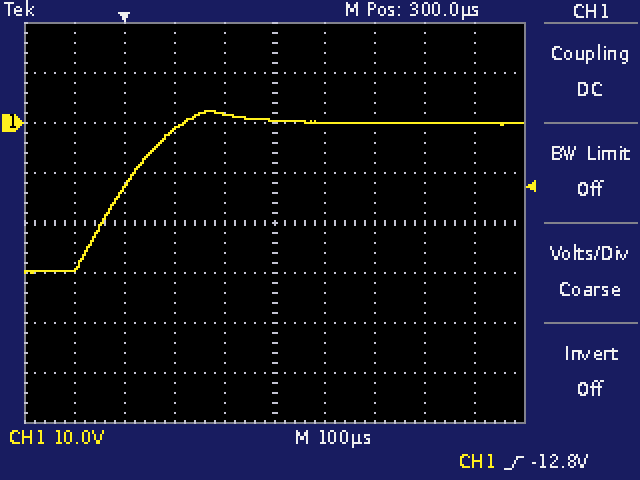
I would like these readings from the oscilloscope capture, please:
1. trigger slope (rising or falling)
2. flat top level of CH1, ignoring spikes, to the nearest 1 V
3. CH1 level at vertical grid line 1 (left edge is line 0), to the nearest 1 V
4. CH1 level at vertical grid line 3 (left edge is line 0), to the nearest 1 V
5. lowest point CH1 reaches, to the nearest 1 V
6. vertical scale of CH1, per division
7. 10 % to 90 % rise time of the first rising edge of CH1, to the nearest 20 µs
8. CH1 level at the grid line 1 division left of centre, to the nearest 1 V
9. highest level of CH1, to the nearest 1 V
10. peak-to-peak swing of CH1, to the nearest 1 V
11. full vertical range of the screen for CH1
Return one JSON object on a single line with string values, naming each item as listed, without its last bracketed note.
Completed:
{"trigger slope": "rising", "flat top level of CH1, ignoring spikes, to the nearest 1 V": "0 V", "CH1 level at vertical grid line 1 (left edge is line 0), to the nearest 1 V": "-29 V", "CH1 level at vertical grid line 3 (left edge is line 0), to the nearest 1 V": "-1 V", "lowest point CH1 reaches, to the nearest 1 V": "-30 V", "vertical scale of CH1, per division": "10 V", "10 % to 90 % rise time of the first rising edge of CH1, to the nearest 20 µs": "160 µs", "CH1 level at the grid line 1 division left of centre, to the nearest 1 V": "2 V", "highest level of CH1, to the nearest 1 V": "2 V", "peak-to-peak swing of CH1, to the nearest 1 V": "32 V", "full vertical range of the screen for CH1": "80 V"}
